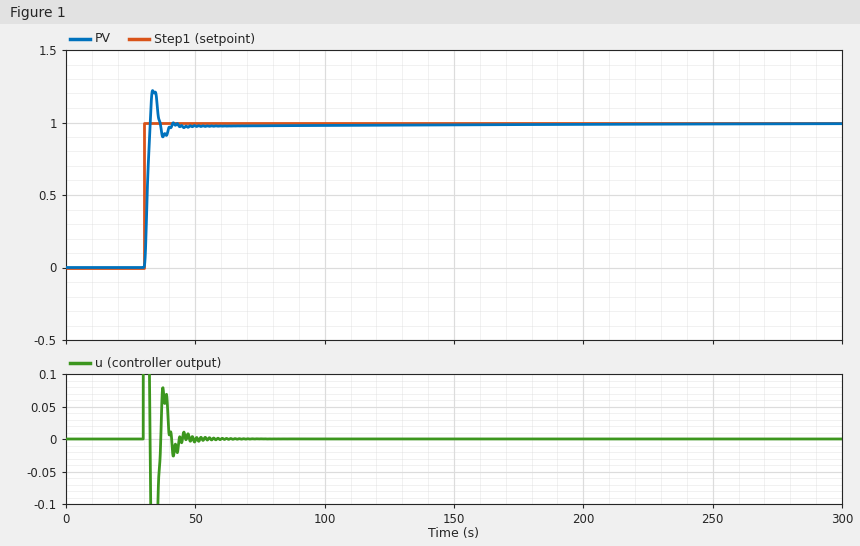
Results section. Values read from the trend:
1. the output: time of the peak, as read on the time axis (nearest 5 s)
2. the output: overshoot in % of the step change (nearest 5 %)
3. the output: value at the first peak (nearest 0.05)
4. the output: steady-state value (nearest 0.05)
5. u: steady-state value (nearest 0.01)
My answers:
35 s
20 %
1.20
1.00
0.00
